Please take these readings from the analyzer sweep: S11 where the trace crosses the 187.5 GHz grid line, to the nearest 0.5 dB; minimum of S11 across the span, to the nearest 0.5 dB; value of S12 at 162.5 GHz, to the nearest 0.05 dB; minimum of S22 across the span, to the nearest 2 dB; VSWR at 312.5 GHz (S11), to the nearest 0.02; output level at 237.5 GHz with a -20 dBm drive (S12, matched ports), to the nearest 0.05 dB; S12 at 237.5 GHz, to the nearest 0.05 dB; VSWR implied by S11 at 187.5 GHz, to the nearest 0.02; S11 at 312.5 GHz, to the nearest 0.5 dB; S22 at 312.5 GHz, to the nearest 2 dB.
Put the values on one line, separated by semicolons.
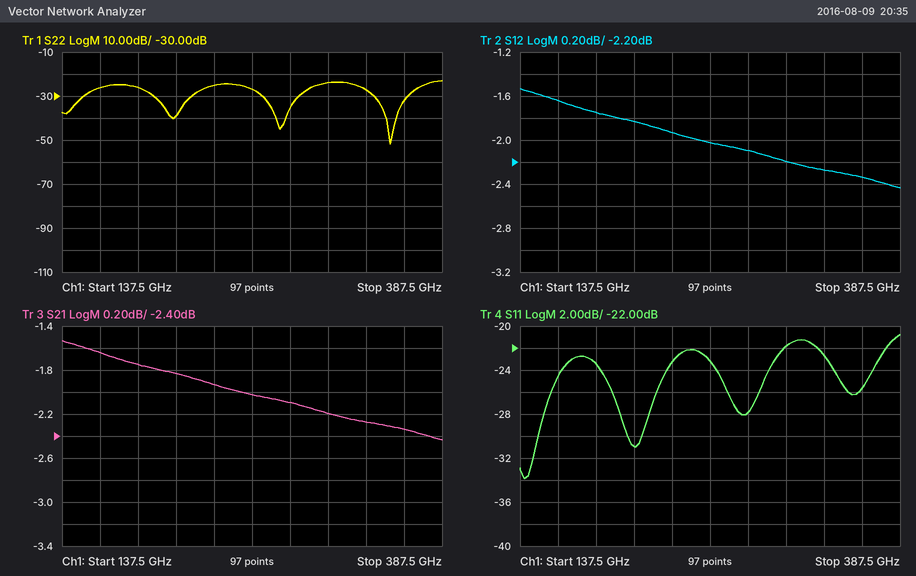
-23.5 dB; -34.0 dB; -1.65 dB; -52 dB; 1.18; -21.95 dBm; -1.95 dB; 1.14; -22.0 dB; -24 dB
